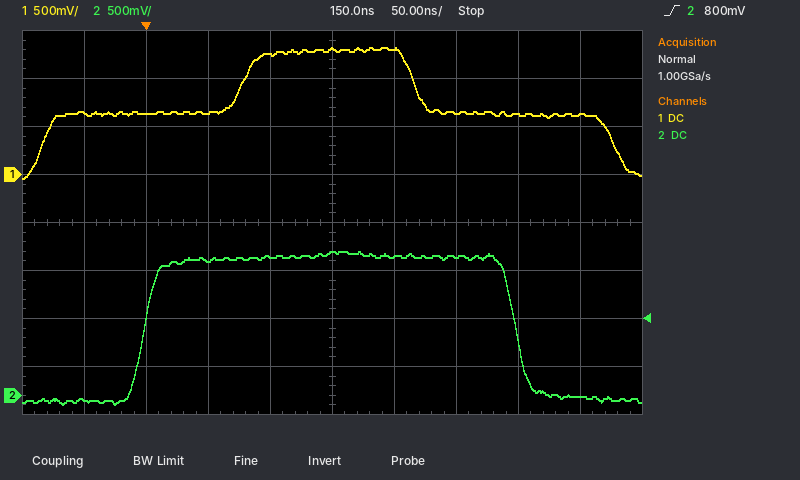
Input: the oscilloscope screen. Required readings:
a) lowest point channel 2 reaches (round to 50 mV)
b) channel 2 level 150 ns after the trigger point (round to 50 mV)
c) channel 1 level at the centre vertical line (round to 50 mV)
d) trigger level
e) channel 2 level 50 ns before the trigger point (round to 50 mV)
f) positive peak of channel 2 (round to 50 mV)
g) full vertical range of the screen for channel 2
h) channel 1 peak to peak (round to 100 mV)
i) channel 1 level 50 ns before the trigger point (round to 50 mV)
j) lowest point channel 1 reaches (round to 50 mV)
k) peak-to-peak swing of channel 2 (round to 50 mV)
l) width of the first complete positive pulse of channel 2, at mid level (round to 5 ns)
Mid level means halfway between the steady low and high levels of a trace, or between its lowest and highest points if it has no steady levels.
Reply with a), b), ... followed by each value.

a) -100 mV
b) 1.50 V
c) 1.30 V
d) 800 mV
e) -50 mV
f) 1.50 V
g) 4 V
h) 1.40 V
i) 650 mV
j) -50 mV
k) 1.60 V
l) 300 ns
